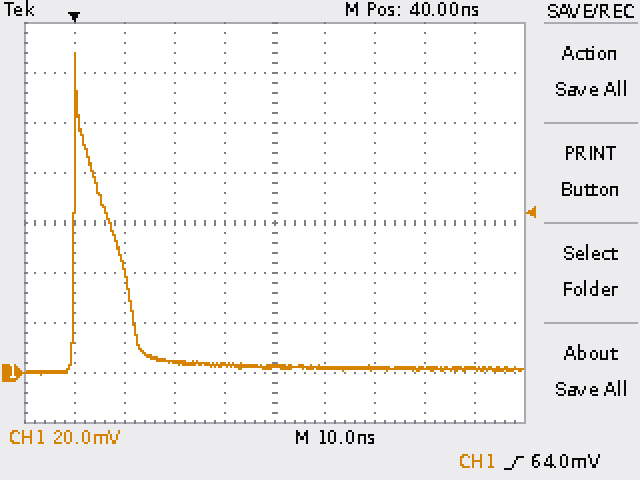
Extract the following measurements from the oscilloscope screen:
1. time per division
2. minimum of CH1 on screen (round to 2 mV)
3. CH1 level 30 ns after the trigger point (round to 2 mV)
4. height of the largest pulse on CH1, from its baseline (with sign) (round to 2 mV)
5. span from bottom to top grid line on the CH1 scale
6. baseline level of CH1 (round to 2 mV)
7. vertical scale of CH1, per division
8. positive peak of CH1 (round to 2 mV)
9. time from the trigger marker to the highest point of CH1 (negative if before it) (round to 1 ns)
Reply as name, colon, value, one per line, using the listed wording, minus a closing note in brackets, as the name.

time per division: 10 ns
minimum of CH1 on screen: 0 mV
CH1 level 30 ns after the trigger point: 4 mV
height of the largest pulse on CH1, from its baseline (with sign): +126 mV
span from bottom to top grid line on the CH1 scale: 160 mV
baseline level of CH1: 2 mV
vertical scale of CH1, per division: 20 mV
positive peak of CH1: 128 mV
time from the trigger marker to the highest point of CH1 (negative if before it): 0 ns
